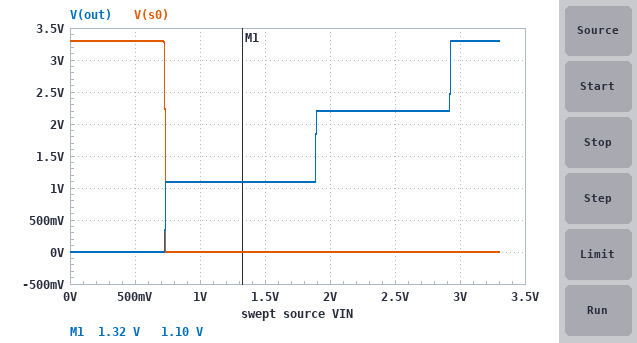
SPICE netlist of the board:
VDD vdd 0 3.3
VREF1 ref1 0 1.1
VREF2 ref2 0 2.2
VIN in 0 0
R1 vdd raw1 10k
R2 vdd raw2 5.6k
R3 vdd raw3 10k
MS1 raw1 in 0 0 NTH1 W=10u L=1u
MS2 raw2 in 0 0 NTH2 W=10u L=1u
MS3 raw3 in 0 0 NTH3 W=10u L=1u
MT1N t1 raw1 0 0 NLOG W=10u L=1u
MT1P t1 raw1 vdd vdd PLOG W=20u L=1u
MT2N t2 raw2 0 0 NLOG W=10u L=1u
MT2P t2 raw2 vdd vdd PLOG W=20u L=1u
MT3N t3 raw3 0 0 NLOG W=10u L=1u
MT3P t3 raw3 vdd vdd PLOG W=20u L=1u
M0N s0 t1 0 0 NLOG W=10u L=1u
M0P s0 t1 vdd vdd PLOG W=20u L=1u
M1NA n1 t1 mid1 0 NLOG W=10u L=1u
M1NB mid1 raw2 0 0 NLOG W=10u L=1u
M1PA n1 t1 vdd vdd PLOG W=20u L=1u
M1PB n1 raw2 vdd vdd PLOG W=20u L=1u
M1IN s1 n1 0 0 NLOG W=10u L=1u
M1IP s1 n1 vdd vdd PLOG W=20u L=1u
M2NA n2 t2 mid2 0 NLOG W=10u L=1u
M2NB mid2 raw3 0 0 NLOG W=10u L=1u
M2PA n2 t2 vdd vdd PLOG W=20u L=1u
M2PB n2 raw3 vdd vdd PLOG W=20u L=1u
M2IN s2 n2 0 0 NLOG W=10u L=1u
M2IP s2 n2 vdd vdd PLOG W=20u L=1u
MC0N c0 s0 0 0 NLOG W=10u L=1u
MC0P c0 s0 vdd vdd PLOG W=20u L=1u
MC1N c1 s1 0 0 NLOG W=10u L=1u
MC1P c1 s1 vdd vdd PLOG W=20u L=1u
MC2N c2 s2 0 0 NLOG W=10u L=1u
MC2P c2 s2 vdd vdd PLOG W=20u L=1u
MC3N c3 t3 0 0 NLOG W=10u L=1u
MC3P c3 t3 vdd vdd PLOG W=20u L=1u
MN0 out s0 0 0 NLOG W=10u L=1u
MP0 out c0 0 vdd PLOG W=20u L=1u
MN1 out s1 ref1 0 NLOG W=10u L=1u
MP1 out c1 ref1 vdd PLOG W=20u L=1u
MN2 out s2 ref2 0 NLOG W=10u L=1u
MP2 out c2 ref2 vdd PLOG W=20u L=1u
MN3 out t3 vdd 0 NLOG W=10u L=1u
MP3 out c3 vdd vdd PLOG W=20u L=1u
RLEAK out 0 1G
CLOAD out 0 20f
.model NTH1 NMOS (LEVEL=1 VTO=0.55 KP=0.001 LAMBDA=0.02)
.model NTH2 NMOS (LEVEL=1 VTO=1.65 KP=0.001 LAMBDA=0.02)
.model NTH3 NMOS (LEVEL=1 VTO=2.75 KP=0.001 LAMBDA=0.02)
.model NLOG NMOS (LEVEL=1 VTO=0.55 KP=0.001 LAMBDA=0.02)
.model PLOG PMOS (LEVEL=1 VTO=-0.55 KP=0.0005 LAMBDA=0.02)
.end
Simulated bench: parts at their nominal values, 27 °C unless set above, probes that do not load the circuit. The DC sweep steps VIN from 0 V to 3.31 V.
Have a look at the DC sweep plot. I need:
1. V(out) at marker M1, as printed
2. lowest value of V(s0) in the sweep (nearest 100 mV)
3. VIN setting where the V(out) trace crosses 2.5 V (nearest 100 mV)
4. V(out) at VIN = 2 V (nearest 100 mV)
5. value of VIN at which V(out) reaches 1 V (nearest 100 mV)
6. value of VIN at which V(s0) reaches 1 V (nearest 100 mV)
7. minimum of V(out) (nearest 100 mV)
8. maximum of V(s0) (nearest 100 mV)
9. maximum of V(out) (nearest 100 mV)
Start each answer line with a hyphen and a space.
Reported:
- 1.10 V
- 0 V
- 2.9 V
- 2.2 V
- 700 mV
- 700 mV
- 0 V
- 3.3 V
- 3.3 V
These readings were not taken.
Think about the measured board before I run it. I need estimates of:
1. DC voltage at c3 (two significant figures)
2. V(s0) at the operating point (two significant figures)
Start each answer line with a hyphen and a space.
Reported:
- 3.3 V
- 3.3 V
